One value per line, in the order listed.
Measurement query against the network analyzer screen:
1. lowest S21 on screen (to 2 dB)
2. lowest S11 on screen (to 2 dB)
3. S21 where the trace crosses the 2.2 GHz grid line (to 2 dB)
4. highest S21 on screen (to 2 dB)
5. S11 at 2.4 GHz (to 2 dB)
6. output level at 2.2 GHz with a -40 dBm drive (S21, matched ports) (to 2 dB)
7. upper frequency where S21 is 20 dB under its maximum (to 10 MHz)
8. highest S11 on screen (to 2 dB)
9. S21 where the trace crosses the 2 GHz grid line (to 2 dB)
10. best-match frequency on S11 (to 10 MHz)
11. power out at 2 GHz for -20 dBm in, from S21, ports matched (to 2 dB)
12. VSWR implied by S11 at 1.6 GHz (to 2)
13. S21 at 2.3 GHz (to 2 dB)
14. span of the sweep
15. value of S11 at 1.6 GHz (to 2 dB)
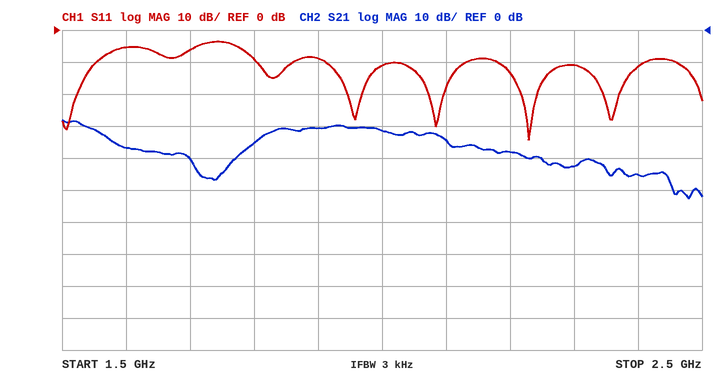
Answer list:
-52 dB
-34 dB
-38 dB
-28 dB
-12 dB
-78 dBm
2.45 GHz
-4 dB
-32 dB
2.23 GHz
-52 dBm
4
-42 dB
1 GHz
-6 dB
